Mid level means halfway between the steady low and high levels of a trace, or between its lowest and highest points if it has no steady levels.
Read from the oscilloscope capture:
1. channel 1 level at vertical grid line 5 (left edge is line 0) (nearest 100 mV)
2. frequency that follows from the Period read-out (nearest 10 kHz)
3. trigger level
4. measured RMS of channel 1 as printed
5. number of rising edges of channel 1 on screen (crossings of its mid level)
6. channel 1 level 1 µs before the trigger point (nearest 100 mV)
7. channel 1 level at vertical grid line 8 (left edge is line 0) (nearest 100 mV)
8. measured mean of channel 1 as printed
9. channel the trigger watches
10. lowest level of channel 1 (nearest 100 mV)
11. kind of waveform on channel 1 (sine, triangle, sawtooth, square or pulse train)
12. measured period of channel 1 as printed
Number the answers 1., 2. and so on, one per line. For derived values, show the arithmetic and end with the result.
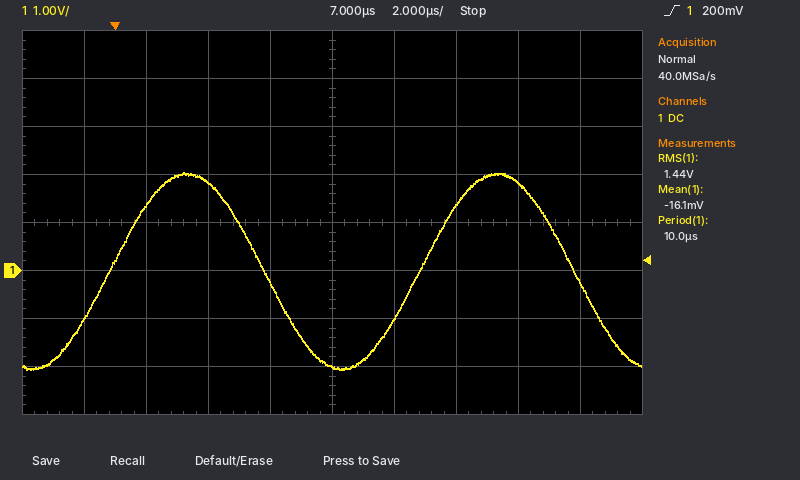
1. -2.0 V
2. 1 / 10.0 µs ≈ 100 kHz
3. 200 mV
4. 1.44 V
5. 2
6. -1.0 V
7. 1.8 V
8. -16.1 mV
9. channel 1
10. -2.1 V
11. sine
12. 10.0 µs
